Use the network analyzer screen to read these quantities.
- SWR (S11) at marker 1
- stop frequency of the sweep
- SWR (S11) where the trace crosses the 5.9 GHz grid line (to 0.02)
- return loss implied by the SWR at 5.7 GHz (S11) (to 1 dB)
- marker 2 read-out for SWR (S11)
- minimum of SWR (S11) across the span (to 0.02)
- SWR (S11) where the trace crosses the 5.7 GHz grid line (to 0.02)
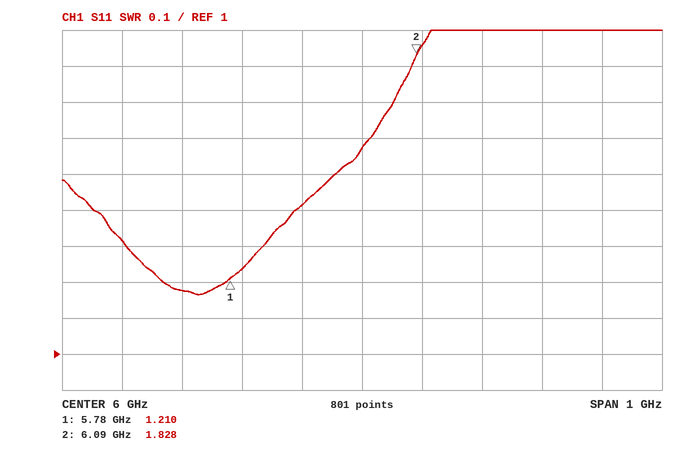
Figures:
1.210
6.5 GHz
1.42
22 dB
1.828
1.16
1.18
